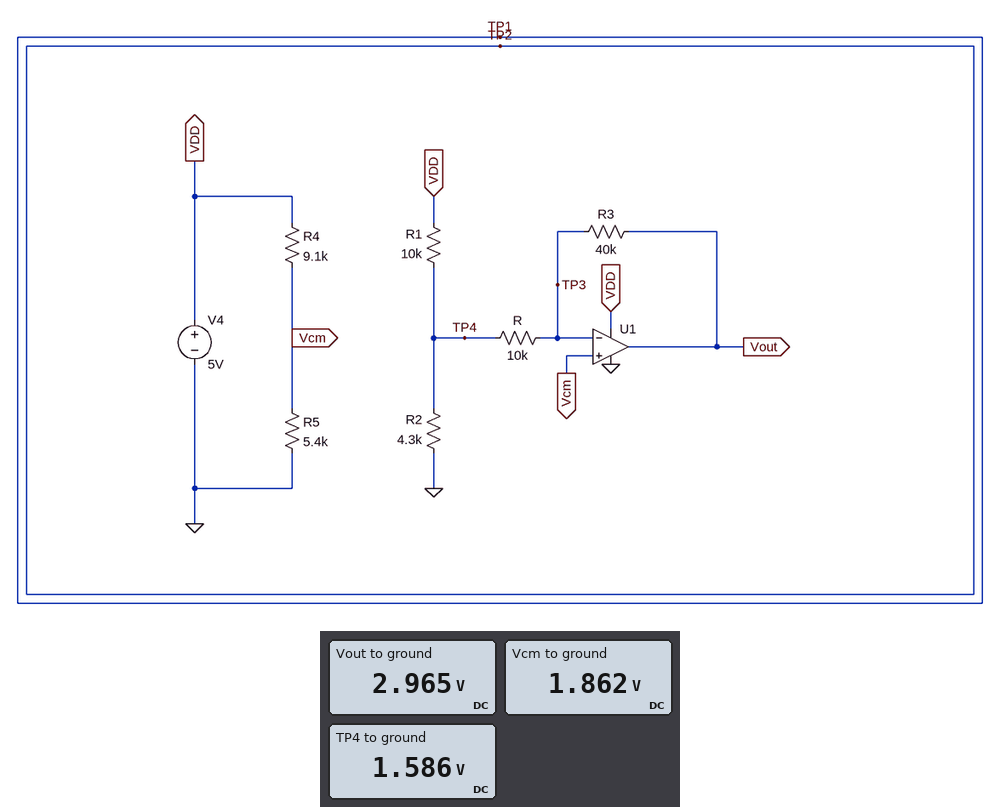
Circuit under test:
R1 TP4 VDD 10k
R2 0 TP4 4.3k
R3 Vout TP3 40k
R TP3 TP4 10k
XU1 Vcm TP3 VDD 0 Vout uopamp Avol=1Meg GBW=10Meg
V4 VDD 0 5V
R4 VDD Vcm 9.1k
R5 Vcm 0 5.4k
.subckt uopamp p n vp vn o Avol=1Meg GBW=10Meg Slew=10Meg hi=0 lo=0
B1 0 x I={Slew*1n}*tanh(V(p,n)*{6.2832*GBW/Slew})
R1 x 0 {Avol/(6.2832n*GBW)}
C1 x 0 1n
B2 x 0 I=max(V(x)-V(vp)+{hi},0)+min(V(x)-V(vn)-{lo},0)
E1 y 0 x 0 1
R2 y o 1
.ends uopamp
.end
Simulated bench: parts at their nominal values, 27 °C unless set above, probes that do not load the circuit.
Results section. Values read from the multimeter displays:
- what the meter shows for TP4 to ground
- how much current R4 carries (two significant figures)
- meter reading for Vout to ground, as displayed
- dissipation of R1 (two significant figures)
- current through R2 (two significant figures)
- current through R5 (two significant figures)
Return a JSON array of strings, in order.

["1.586 V", "340 µA", "2.965 V", "1.2 mW", "370 µA", "340 µA"]
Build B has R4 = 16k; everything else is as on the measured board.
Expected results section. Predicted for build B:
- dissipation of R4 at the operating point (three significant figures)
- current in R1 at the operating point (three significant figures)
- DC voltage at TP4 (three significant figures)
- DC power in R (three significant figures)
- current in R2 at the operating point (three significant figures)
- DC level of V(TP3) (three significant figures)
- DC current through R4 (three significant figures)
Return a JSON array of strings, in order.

["873 µW", "355 µA", "1.45 V", "3.46 µW", "337 µA", "1.26 V", "234 µA"]
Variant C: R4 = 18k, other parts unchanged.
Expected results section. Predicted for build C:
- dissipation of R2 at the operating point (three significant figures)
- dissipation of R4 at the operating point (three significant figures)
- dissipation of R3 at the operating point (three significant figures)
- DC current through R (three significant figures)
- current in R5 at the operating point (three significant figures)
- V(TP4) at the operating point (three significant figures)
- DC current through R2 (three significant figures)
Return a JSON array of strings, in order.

["471 µW", "822 µW", "28.9 µW", "26.9 µA", "214 µA", "1.42 V", "331 µA"]
